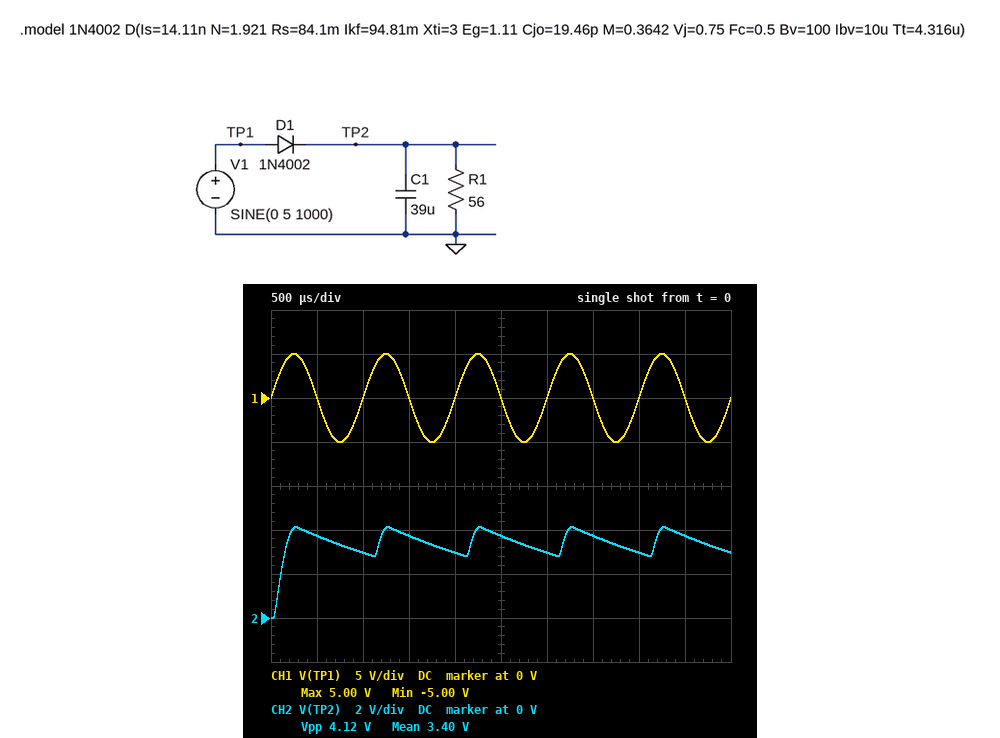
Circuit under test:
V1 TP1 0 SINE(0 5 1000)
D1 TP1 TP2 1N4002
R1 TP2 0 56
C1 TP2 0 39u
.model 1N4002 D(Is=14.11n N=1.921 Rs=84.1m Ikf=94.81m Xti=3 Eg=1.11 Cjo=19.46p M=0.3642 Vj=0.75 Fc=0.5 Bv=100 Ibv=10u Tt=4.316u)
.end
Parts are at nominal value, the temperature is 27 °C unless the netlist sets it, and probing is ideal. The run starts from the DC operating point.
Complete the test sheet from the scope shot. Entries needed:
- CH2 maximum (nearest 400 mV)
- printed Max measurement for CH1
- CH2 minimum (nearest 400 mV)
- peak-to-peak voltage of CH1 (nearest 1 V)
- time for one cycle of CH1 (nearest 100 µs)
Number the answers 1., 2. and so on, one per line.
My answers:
1. 4.0 V
2. 5.00 V
3. 0 V
4. 10 V
5. 1.0 ms
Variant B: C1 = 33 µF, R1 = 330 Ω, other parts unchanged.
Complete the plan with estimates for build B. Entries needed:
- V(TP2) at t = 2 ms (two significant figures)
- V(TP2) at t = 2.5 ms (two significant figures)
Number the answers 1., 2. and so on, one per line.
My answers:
1. 3.9 V
2. 4.1 V
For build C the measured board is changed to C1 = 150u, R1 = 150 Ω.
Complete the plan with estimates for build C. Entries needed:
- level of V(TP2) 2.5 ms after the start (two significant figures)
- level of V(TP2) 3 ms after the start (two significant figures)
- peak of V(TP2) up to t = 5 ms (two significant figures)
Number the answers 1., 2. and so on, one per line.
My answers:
1. 4.0 V
2. 3.9 V
3. 4.1 V
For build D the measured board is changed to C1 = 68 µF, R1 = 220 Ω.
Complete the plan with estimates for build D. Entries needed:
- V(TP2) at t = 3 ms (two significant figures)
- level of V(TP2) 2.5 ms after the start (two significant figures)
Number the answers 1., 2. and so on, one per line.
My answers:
1. 3.9 V
2. 4.1 V
